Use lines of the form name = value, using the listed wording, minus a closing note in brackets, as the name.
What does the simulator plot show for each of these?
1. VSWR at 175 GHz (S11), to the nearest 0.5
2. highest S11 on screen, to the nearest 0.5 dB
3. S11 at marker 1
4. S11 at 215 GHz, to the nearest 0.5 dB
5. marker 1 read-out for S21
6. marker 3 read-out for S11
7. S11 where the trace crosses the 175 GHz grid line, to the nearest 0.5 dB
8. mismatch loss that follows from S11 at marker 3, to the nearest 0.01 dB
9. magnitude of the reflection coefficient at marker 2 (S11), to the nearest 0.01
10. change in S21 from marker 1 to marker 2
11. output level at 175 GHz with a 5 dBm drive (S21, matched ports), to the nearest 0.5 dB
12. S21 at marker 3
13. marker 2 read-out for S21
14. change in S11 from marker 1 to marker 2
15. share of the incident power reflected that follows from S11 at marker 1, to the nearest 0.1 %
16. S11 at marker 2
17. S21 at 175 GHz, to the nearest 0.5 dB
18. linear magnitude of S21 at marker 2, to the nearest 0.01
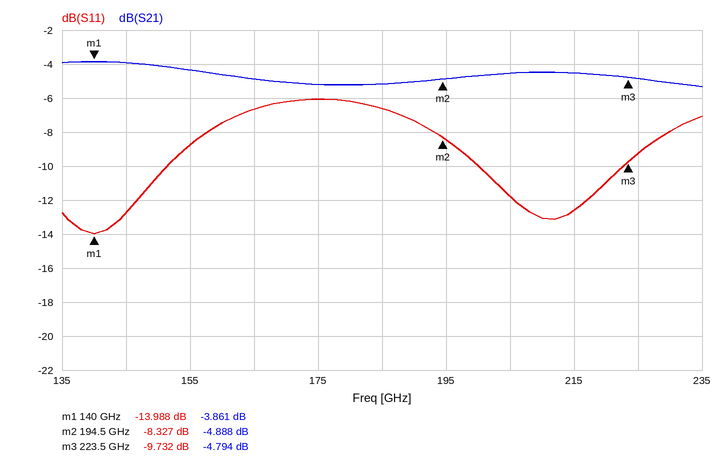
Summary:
VSWR at 175 GHz (S11), to the nearest 0.5 = 3.0
highest S11 on screen, to the nearest 0.5 dB = -6.0 dB
S11 at marker 1 = -13.988 dB
S11 at 215 GHz, to the nearest 0.5 dB = -12.5 dB
marker 1 read-out for S21 = -3.861 dB
marker 3 read-out for S11 = -9.732 dB
S11 where the trace crosses the 175 GHz grid line, to the nearest 0.5 dB = -6.0 dB
mismatch loss that follows from S11 at marker 3, to the nearest 0.01 dB = 0.49 dB
magnitude of the reflection coefficient at marker 2 (S11), to the nearest 0.01 = 0.38
change in S21 from marker 1 to marker 2 = -1.027 dB
output level at 175 GHz with a 5 dBm drive (S21, matched ports), to the nearest 0.5 dB = 0.0 dBm
S21 at marker 3 = -4.794 dB
marker 2 read-out for S21 = -4.888 dB
change in S11 from marker 1 to marker 2 = 5.661 dB
share of the incident power reflected that follows from S11 at marker 1, to the nearest 0.1 % = 4.0 %
S11 at marker 2 = -8.327 dB
S21 at 175 GHz, to the nearest 0.5 dB = -5.0 dB
linear magnitude of S21 at marker 2, to the nearest 0.01 = 0.57
